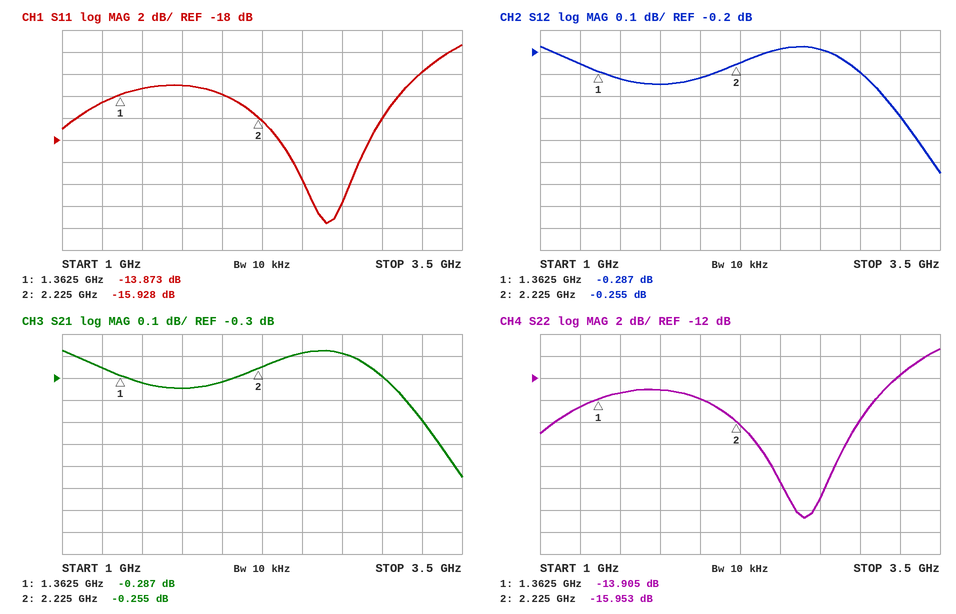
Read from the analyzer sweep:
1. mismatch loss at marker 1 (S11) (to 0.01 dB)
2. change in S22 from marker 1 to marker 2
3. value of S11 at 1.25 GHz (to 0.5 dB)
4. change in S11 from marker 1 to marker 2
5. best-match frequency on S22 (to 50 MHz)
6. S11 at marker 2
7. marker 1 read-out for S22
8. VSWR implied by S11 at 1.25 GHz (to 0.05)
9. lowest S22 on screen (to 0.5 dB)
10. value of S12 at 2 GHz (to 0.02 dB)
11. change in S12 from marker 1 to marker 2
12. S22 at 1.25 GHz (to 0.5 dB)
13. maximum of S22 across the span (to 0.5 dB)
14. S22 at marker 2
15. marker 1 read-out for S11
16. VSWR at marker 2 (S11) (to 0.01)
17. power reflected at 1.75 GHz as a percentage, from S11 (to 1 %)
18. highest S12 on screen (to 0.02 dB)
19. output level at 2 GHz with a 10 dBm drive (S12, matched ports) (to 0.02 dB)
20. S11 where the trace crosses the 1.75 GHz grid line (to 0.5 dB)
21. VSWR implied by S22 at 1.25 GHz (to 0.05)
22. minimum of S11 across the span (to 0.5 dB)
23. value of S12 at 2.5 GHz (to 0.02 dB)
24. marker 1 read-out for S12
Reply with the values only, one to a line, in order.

0.18 dB
-2.048 dB
-14.5 dB
-2.055 dB
2.65 GHz
-15.928 dB
-13.905 dB
1.45
-24.5 dB
-0.32 dB
0.032 dB
-14.5 dB
-9.5 dB
-15.953 dB
-13.873 dB
1.38
5 %
-0.18 dB
9.68 dBm
-13.0 dB
1.45
-25.5 dB
-0.18 dB
-0.287 dB
